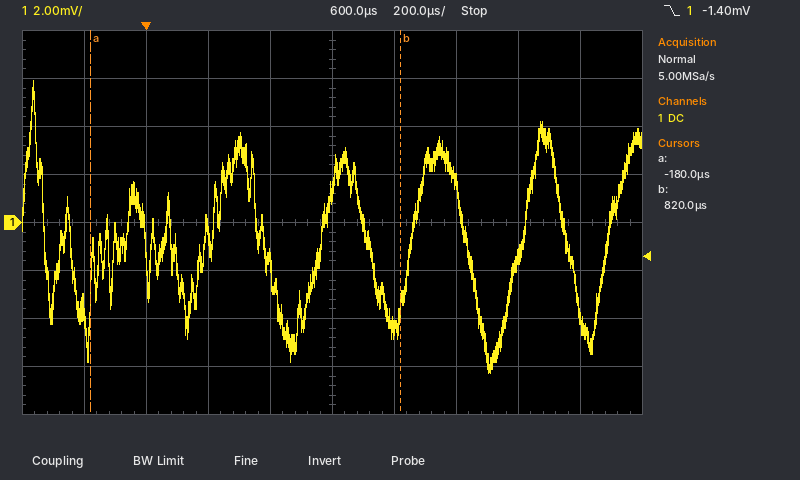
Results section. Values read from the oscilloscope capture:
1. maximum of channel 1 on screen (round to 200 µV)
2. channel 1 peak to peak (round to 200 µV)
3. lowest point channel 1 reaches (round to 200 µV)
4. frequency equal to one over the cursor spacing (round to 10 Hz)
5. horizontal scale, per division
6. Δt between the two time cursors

6.0 mV
12.2 mV
-6.2 mV
1.00 kHz
200 µs
1.00 ms
